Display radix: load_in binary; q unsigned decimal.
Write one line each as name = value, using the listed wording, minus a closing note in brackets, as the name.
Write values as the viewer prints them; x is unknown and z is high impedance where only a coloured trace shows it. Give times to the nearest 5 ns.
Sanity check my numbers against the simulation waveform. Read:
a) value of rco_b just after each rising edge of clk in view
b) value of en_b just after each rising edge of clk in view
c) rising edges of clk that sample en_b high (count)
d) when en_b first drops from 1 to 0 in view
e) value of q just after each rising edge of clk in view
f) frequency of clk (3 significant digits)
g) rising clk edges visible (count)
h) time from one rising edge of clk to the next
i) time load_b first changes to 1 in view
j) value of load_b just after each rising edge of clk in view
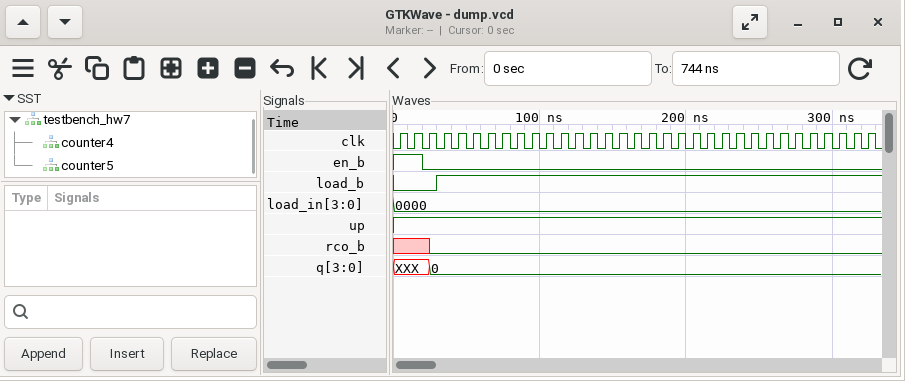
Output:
value of rco_b just after each rising edge of clk in view = x x 0 0 0 0 0 0 0 0 0 0 0 0 0 0 0 0 0 0 0 0 0 0 0 0 0 0 0 0 0 0 0
value of en_b just after each rising edge of clk in view = 1 1 0 0 0 0 0 0 0 0 0 0 0 0 0 0 0 0 0 0 0 0 0 0 0 0 0 0 0 0 0 0 0
rising edges of clk that sample en_b high = 2
when en_b first drops from 1 to 0 in view = 20 ns
value of q just after each rising edge of clk in view = XXX, XXX, 0, 0, 0, 0, 0, 0, 0, 0, 0, 0, 0, 0, 0, 0, 0, 0, 0, 0, 0, 0, 0, 0, 0, 0, 0, 0, 0, 0, 0, 0, 0
frequency of clk = 100 MHz
rising clk edges visible = 33
time from one rising edge of clk to the next = 10 ns
time load_b first changes to 1 in view = 30 ns
value of load_b just after each rising edge of clk in view = 0 0 0 1 1 1 1 1 1 1 1 1 1 1 1 1 1 1 1 1 1 1 1 1 1 1 1 1 1 1 1 1 1
